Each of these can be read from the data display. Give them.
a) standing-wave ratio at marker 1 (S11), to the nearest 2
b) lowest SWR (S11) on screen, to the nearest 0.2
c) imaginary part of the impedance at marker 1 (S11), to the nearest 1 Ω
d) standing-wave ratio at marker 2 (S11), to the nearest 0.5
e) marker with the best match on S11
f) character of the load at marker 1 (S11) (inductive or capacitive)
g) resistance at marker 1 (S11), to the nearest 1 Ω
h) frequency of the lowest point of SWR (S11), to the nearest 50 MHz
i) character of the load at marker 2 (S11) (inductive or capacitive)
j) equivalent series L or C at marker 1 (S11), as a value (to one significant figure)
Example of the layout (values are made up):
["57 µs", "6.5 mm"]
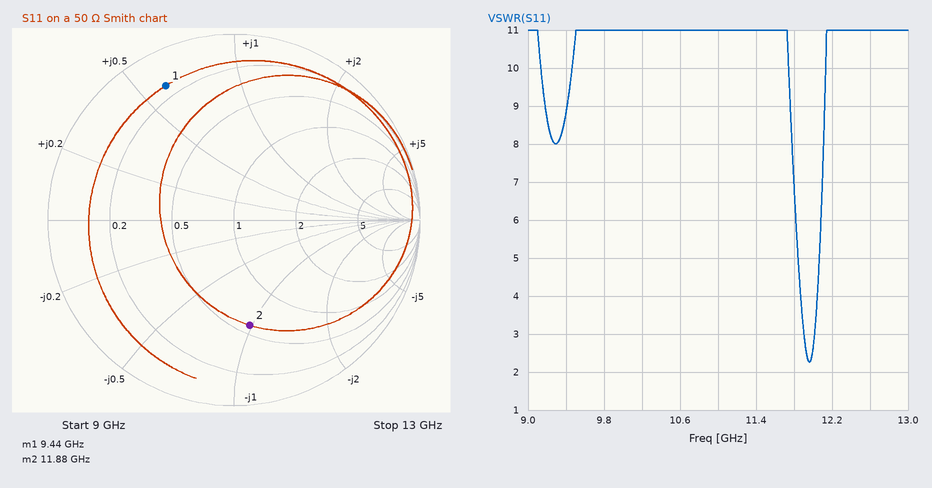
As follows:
["10", "2.2", "+30 Ω", "3.5", "marker 2", "inductive", "7 Ω", "11.95 GHz", "capacitive", "500 pH"]
